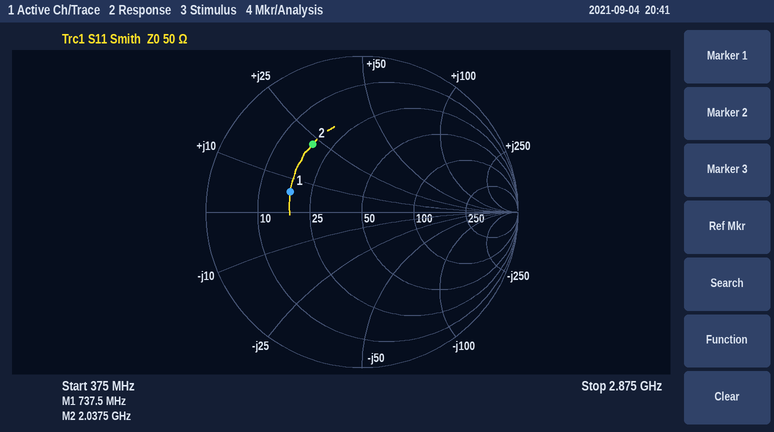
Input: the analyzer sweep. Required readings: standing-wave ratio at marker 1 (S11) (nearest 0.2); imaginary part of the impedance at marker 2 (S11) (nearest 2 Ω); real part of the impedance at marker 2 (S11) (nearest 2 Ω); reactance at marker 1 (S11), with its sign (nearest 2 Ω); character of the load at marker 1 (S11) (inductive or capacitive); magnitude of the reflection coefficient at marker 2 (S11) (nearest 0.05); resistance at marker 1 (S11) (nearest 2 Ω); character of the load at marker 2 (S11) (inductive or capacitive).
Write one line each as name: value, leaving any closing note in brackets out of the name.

standing-wave ratio at marker 1 (S11): 2.8
imaginary part of the impedance at marker 2 (S11): +22 Ω
real part of the impedance at marker 2 (S11): 18 Ω
reactance at marker 1 (S11), with its sign: +6 Ω
character of the load at marker 1 (S11): inductive
magnitude of the reflection coefficient at marker 2 (S11): 0.55
resistance at marker 1 (S11): 18 Ω
character of the load at marker 2 (S11): inductive
